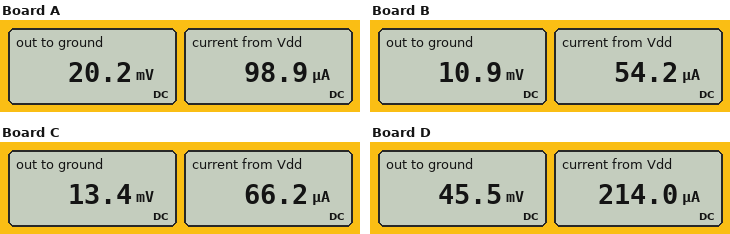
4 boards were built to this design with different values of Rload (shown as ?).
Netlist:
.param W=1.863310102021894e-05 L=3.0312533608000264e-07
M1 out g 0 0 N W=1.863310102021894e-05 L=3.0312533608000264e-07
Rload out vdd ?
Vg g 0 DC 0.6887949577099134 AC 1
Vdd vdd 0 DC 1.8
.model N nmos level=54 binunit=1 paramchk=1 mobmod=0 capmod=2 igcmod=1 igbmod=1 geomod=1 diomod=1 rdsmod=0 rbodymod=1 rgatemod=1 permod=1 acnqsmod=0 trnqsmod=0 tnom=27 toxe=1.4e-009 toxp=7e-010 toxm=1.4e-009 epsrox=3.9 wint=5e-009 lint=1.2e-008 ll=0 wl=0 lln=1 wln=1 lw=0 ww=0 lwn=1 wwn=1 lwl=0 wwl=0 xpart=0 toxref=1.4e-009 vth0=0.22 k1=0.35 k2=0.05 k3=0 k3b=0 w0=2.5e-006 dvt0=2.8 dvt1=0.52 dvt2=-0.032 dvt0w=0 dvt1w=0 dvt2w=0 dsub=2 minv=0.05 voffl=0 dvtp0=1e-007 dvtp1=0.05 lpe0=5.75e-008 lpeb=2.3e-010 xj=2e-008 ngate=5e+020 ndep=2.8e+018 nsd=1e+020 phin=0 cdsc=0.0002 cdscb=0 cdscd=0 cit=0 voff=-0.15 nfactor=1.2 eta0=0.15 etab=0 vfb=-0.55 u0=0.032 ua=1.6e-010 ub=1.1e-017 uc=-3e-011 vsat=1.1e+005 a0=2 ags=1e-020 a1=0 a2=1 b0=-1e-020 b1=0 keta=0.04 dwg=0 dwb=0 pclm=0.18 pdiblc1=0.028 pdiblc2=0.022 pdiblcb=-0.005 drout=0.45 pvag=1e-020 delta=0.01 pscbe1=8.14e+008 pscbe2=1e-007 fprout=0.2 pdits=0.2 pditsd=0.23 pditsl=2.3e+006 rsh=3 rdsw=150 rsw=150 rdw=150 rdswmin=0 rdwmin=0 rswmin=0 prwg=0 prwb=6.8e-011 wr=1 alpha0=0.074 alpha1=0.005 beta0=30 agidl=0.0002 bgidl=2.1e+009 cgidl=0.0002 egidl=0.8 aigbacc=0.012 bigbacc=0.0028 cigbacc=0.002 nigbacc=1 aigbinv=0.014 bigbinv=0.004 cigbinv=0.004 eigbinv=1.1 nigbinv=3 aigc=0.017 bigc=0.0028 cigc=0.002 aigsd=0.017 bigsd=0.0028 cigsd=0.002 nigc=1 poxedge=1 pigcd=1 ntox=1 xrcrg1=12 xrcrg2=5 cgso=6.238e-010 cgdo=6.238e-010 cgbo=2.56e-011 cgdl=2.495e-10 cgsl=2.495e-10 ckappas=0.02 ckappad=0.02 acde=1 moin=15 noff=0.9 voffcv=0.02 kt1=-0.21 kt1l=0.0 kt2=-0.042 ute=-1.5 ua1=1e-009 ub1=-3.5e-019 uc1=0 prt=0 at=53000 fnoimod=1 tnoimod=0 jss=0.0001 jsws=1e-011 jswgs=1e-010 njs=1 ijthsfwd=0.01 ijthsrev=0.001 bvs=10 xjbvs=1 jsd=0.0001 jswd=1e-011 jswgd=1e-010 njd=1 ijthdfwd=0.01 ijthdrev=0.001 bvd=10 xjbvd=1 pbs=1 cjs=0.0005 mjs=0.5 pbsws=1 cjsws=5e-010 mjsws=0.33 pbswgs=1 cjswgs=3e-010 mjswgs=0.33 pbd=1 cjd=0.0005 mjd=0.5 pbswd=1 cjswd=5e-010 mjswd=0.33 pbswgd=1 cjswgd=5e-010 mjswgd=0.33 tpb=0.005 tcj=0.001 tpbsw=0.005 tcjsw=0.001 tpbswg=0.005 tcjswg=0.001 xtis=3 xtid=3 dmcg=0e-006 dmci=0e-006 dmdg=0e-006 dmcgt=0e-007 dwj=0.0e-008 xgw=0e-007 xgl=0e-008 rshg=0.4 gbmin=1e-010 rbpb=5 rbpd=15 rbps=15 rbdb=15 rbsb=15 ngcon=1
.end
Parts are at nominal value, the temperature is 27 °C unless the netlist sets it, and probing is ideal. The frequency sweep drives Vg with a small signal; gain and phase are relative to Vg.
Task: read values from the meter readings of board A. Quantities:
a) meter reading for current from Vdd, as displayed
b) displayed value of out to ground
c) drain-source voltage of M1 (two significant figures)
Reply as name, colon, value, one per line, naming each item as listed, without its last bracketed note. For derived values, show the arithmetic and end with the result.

meter reading for current from Vdd, as displayed: 98.9 µA
displayed value of out to ground: 20.2 mV
drain-source voltage of M1: 20.2 mV = 20 mV
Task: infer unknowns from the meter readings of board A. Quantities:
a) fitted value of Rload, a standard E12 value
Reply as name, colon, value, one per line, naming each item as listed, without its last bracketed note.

fitted value of Rload, a standard E12 value: 18 kΩ
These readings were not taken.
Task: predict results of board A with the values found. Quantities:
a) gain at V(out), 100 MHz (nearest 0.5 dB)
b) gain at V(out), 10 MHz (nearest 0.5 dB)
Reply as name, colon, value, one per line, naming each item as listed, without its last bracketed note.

gain at V(out), 100 MHz: -32.0 dB
gain at V(out), 10 MHz: -33.5 dB
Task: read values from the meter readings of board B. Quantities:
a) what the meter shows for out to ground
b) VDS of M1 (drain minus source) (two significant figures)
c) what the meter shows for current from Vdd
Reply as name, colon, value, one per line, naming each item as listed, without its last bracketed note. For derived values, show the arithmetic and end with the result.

what the meter shows for out to ground: 10.9 mV
VDS of M1 (drain minus source): 10.9 mV = 11 mV
what the meter shows for current from Vdd: 54.2 µA
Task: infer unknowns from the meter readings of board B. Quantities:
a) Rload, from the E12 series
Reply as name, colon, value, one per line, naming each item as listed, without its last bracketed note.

Rload, from the E12 series: 33 kΩ
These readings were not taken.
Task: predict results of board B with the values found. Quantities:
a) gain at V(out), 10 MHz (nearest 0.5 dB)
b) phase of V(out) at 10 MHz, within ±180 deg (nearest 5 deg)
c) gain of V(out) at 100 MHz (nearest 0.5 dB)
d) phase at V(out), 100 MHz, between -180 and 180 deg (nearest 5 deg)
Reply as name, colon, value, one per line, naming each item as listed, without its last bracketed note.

gain at V(out), 10 MHz: -39.5 dB
phase of V(out) at 10 MHz, within ±180 deg: 170 deg
gain of V(out) at 100 MHz: -35.0 dB
phase at V(out), 100 MHz, between -180 and 180 deg: 125 deg
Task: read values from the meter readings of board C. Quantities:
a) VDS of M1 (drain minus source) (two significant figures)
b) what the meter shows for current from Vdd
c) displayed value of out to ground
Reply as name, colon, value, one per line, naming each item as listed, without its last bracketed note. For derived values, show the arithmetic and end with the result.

VDS of M1 (drain minus source): 13.4 mV = 13 mV
what the meter shows for current from Vdd: 66.2 µA
displayed value of out to ground: 13.4 mV
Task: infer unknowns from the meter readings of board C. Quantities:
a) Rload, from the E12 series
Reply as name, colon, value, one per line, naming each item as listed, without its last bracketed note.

Rload, from the E12 series: 27 kΩ
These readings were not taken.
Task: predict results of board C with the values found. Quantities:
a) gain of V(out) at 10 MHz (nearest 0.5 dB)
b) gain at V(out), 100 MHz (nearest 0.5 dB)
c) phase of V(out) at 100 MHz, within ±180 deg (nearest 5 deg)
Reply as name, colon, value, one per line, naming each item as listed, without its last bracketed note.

gain of V(out) at 10 MHz: -37.5 dB
gain at V(out), 100 MHz: -34.0 dB
phase of V(out) at 100 MHz, within ±180 deg: 130 deg
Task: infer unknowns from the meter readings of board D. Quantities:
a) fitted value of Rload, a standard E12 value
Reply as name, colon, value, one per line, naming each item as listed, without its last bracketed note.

fitted value of Rload, a standard E12 value: 8.2 kΩ
